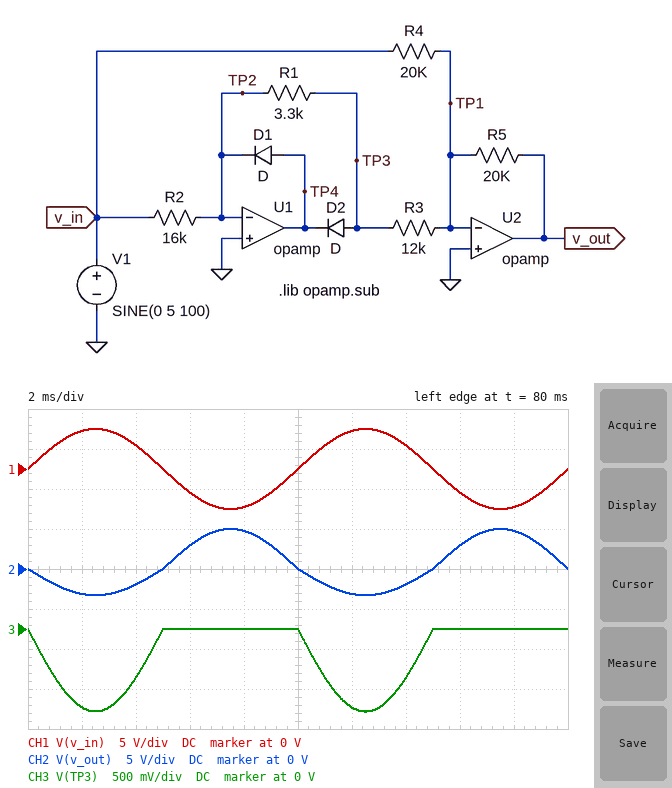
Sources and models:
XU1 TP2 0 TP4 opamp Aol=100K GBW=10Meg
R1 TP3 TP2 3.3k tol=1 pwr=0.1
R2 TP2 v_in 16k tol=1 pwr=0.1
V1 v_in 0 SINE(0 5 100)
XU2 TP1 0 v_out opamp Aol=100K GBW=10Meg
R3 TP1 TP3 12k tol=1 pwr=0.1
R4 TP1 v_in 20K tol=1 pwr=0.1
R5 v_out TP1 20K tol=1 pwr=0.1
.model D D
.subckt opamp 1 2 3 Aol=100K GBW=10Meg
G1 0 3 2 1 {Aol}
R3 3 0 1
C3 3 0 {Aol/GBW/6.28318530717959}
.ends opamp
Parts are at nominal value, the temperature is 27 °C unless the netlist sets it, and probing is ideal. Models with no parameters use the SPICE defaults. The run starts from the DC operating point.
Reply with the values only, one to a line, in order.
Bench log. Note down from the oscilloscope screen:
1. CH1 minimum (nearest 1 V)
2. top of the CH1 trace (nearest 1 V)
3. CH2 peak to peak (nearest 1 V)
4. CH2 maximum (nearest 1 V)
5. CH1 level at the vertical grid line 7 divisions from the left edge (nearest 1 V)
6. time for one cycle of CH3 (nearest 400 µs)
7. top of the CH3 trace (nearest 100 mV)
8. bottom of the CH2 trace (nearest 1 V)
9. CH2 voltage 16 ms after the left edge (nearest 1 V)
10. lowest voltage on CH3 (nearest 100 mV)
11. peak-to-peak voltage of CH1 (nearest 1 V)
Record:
-5 V
5 V
8 V
5 V
3 V
10.0 ms
0 V
-3 V
3 V
-1.0 V
10 V
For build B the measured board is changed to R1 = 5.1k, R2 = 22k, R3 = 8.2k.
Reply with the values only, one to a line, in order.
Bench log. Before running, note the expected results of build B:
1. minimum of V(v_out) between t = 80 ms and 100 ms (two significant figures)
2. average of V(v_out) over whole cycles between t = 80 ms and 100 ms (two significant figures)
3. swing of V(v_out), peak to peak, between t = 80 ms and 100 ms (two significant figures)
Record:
-2.2 V
900 mV
7.2 V
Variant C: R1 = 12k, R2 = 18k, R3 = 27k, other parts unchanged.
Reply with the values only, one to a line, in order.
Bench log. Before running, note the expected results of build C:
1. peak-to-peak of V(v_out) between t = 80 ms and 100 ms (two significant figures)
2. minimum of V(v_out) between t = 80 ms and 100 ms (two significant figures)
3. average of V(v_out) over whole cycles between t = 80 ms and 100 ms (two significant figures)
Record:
7.5 V
-2.5 V
790 mV
